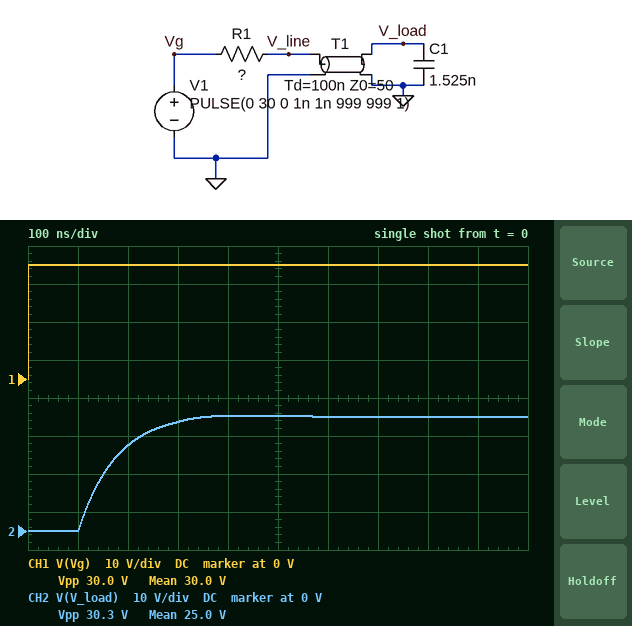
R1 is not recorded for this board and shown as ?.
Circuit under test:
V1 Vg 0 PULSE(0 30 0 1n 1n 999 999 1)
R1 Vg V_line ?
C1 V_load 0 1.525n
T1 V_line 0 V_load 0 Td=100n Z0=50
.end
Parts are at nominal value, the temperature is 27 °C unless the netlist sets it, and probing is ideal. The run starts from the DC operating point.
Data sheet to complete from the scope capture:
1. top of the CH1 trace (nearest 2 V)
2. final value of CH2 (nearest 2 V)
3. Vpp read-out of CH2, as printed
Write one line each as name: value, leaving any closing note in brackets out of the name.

top of the CH1 trace: 30 V
final value of CH2: 30 V
Vpp read-out of CH2, as printed: 30.3 V
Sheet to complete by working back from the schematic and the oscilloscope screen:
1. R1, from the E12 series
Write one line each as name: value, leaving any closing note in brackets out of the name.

R1, from the E12 series: 47 Ω
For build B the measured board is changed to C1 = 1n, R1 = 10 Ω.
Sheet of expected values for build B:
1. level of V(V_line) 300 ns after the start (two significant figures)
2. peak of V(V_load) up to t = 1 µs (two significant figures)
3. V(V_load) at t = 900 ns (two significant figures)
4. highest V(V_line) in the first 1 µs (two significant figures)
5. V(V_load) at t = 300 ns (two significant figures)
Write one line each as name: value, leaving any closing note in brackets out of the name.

level of V(V_line) 300 ns after the start: 31 V
peak of V(V_load) up to t = 1 µs: 57 V
V(V_load) at t = 900 ns: 40 V
highest V(V_line) in the first 1 µs: 36 V
V(V_load) at t = 300 ns: 49 V
